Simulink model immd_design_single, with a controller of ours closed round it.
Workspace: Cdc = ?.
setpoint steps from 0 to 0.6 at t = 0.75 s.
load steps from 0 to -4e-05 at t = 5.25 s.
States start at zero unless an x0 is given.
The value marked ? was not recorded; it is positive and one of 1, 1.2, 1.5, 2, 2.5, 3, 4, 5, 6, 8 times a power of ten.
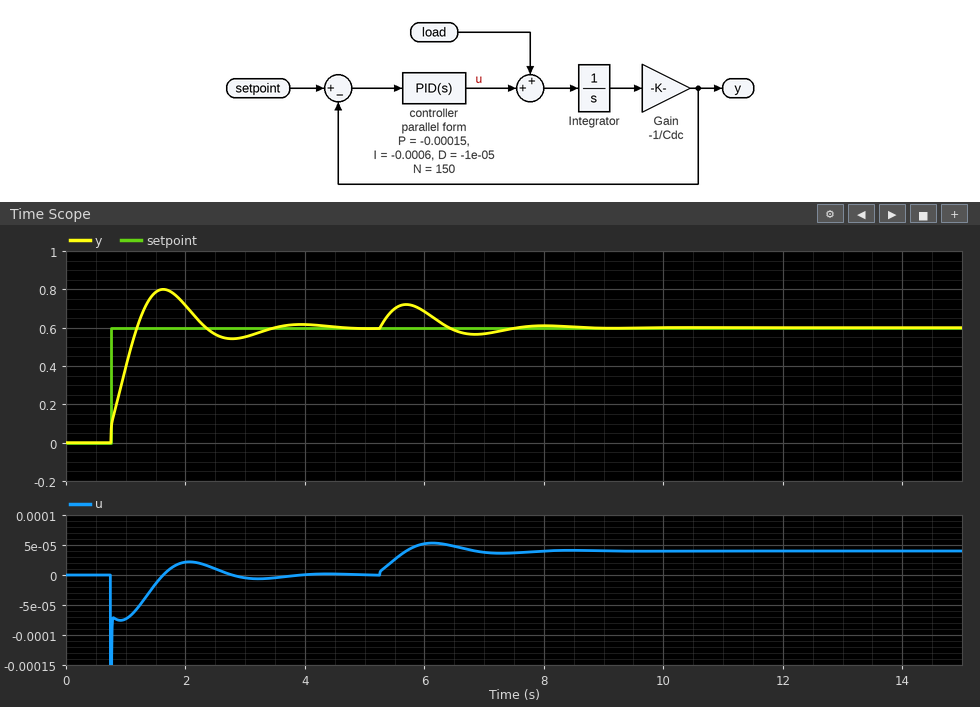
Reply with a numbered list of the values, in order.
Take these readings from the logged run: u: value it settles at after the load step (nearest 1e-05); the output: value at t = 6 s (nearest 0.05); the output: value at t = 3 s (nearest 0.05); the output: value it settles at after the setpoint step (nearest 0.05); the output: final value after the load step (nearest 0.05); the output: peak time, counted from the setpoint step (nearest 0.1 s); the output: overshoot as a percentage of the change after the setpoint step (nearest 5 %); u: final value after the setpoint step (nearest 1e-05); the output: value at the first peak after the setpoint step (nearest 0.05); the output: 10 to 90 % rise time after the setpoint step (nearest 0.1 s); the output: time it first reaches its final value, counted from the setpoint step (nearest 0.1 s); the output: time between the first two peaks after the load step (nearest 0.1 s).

1. 0.00004
2. 0.70
3. 0.55
4. 0.60
5. 0.60
6. 0.9 s
7. 35 %
8. 0.00000
9. 0.80
10. 0.4 s
11. 0.4 s
12. 2.3 s
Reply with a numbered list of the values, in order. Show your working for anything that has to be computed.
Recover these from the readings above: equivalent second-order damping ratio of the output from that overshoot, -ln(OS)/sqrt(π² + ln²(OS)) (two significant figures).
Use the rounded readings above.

1. ln(0.35) = -1.050; 1.050 / sqrt(9.870 + 1.102) = 0.32
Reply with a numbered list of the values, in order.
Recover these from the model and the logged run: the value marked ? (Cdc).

1. 6e-05
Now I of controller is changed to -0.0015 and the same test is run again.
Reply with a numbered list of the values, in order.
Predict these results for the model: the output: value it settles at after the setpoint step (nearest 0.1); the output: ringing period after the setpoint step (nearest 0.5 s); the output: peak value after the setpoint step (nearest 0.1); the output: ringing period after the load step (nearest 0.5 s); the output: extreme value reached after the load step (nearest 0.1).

1. 0.6
2. 1.5 s
3. 0.9
4. 1.5 s
5. 0.7
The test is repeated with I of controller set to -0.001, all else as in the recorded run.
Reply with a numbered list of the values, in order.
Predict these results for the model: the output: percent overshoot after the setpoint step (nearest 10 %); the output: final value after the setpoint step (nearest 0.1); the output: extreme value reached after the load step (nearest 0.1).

1. 40 %
2. 0.6
3. 0.7
